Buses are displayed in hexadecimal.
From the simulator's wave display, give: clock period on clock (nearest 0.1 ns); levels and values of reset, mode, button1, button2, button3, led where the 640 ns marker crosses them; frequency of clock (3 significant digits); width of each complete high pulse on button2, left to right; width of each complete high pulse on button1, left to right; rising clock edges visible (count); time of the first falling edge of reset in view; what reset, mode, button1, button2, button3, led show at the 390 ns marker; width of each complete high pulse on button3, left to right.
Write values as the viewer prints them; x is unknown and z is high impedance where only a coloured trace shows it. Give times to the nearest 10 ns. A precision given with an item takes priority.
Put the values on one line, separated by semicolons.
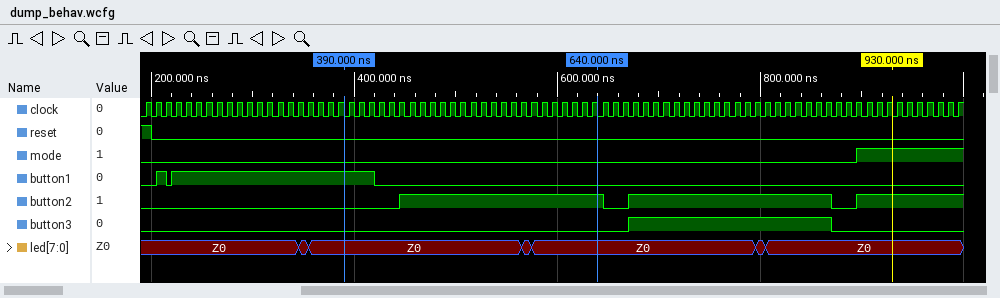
10 ns; reset=0, mode=0, button1=0, button2=1, button3=0, led=Z0; 100 MHz; 200 ns, 200 ns; 10 ns, 200 ns; 81; 200 ns; reset=0, mode=0, button1=1, button2=0, button3=0, led=Z0; 200 ns
